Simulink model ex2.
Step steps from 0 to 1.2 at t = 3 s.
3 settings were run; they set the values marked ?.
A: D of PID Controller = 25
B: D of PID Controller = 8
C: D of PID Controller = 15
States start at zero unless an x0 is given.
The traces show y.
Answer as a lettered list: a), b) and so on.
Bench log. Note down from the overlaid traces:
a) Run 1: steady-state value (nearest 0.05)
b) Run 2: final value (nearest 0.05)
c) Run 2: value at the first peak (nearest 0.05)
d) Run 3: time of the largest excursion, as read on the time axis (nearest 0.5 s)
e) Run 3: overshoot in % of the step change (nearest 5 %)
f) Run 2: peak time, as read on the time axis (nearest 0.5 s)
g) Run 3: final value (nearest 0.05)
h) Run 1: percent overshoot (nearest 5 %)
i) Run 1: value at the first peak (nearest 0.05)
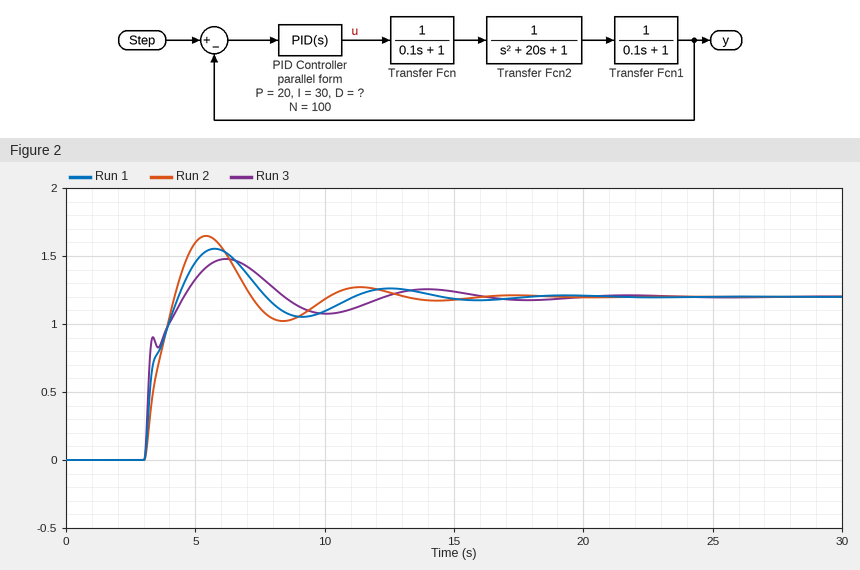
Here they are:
a) 1.20
b) 1.20
c) 1.65
d) 6.0 s
e) 25 %
f) 5.5 s
g) 1.20
h) 30 %
i) 1.55
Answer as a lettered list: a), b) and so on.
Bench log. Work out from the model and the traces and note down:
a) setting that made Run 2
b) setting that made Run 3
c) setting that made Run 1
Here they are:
a) B
b) A
c) C
